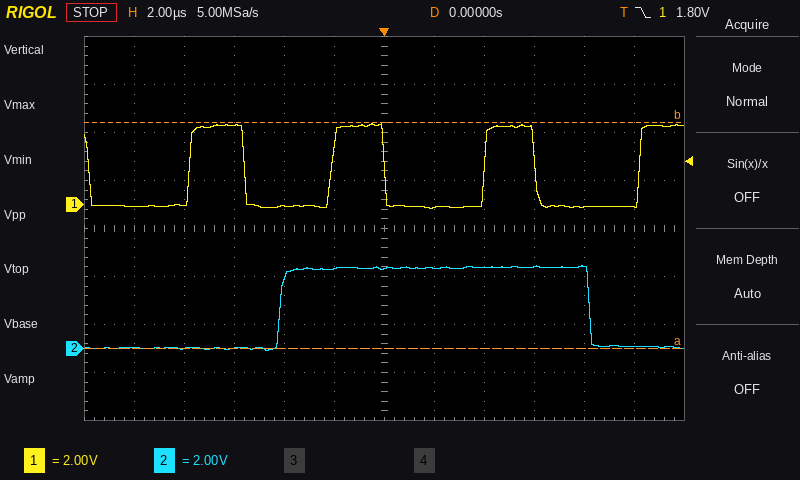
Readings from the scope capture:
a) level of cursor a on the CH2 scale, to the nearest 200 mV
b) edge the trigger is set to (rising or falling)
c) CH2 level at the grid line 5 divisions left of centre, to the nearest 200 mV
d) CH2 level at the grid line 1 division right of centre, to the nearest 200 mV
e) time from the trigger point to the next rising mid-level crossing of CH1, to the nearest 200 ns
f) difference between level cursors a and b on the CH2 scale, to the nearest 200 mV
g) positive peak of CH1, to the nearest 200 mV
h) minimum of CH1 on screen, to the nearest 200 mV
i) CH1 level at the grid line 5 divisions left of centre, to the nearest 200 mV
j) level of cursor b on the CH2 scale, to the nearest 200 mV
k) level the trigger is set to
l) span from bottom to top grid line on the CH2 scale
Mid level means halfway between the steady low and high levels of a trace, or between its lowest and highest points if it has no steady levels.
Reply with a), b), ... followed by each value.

a) 0.0 V
b) falling
c) 0.0 V
d) 3.4 V
e) 4.0 µs
f) 9.4 V
g) 3.4 V
h) -200 mV
i) 0.0 V
j) 9.4 V
k) 1.80 V
l) 16 V
